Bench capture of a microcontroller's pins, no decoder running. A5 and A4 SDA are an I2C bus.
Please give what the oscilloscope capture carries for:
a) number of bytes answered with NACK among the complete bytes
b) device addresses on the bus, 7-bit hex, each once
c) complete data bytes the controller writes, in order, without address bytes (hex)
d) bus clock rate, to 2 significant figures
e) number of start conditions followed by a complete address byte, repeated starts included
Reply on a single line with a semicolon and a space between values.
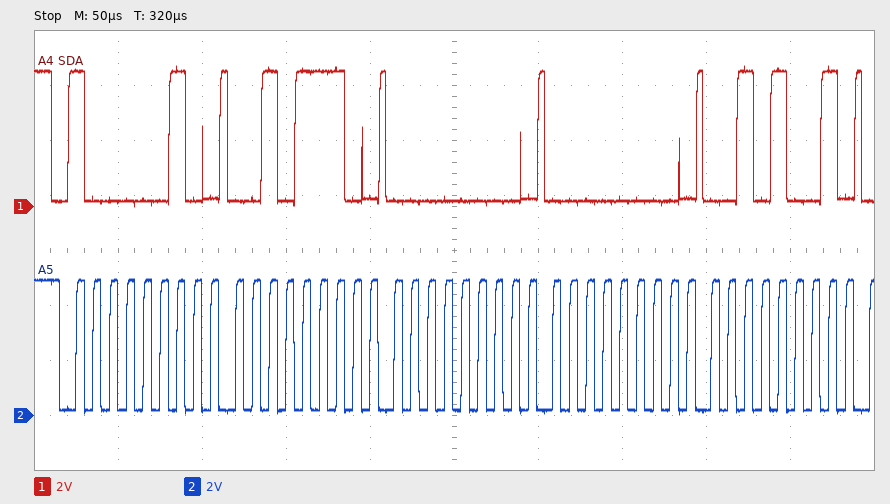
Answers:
0; 0x41; 2E 00 00 29; 100 kHz; 1
